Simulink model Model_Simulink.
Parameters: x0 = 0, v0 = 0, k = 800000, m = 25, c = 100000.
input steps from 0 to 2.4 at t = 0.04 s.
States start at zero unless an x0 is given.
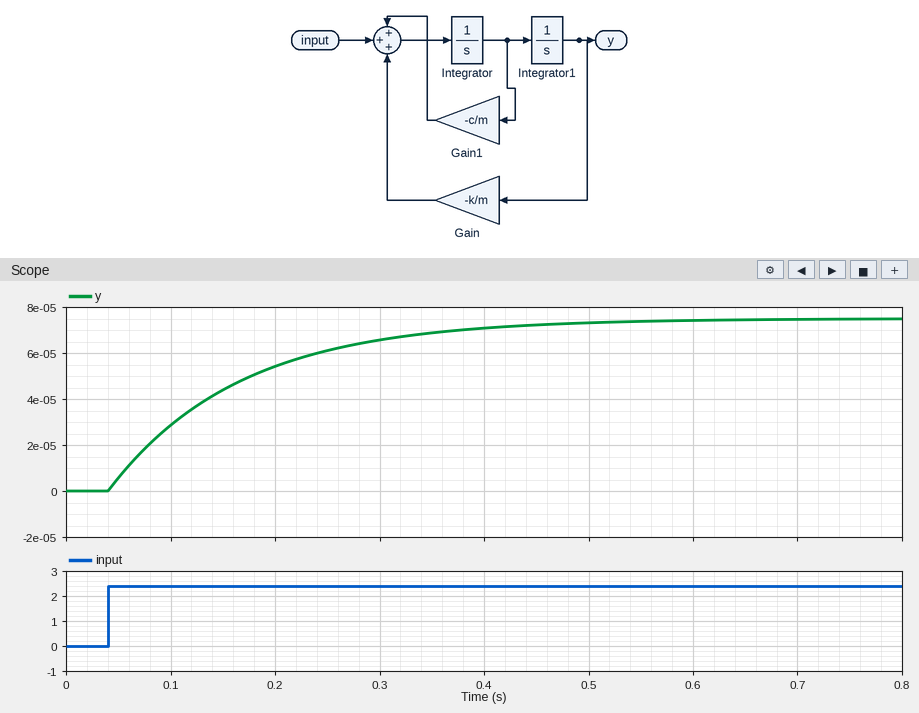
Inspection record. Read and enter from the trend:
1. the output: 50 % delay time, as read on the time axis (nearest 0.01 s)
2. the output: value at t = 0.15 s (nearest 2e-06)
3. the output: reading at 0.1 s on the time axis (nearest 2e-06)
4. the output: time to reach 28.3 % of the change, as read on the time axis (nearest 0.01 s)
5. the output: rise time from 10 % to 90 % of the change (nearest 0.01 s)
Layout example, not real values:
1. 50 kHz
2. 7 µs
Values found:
1. 0.13 s
2. 0.000044
3. 0.000028
4. 0.08 s
5. 0.27 s
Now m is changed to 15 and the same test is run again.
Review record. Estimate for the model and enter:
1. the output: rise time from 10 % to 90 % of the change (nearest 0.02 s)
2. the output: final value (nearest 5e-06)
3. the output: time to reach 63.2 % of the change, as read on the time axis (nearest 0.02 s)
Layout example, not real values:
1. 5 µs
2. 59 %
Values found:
1. 0.28 s
2. 0.000045
3. 0.16 s
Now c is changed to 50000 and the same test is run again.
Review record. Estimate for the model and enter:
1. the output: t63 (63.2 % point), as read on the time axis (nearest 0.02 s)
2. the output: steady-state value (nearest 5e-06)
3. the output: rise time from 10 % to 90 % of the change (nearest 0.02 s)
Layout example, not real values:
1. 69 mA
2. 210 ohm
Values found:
1. 0.10 s
2. 0.000075
3. 0.14 s
